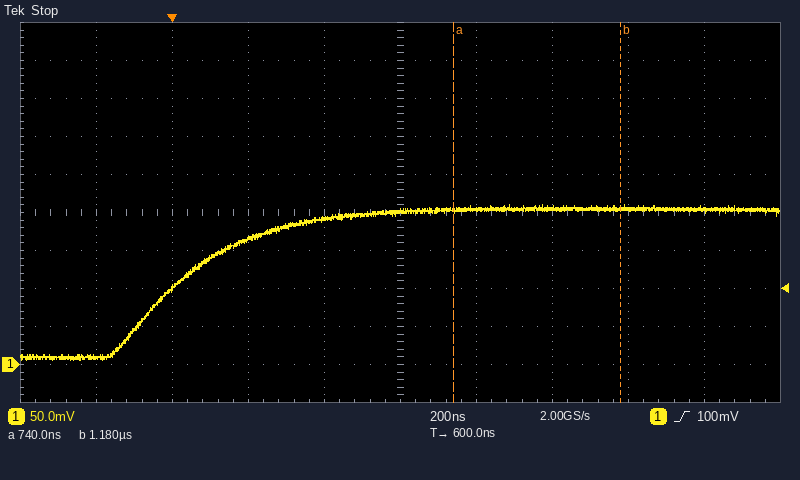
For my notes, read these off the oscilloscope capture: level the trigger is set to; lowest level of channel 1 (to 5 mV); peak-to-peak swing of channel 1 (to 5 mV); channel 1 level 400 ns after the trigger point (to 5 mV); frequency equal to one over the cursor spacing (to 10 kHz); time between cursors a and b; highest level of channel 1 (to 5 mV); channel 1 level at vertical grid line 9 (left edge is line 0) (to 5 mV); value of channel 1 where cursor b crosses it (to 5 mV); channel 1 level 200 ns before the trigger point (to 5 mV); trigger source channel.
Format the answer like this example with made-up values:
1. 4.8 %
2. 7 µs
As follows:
1. 100 mV
2. 5 mV
3. 205 mV
4. 190 mV
5. 2.27 MHz
6. 440 ns
7. 210 mV
8. 205 mV
9. 205 mV
10. 10 mV
11. channel 1
